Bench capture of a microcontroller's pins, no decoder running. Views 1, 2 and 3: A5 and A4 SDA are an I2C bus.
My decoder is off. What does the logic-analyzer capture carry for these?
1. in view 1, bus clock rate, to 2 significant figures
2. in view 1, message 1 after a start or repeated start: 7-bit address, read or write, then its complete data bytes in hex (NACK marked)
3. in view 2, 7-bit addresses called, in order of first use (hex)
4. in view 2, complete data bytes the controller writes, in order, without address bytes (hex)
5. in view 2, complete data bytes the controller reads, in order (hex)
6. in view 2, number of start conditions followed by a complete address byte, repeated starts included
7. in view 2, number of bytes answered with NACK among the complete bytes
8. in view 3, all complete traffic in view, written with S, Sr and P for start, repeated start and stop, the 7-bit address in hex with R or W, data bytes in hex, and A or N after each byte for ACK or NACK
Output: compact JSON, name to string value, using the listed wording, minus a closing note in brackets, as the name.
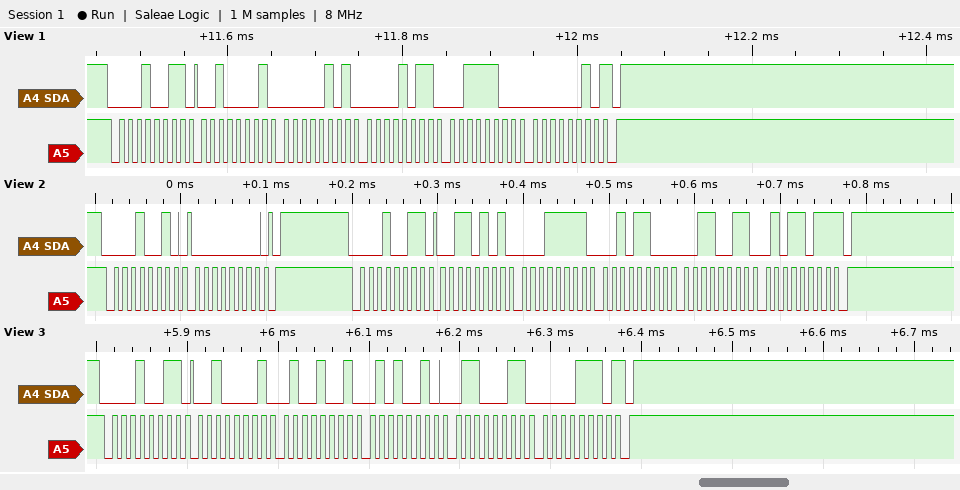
{"in view 1, bus clock rate, to 2 significant figures": "100 kHz", "in view 1, message 1 after a start or repeated start: 7-bit address, read or write, then its complete data bytes in hex": "0x09 read: 21 05 0B 3C 02 NACK", "in view 2, 7-bit addresses called, in order of first use": "0x09", "in view 2, complete data bytes the controller writes, in order, without address bytes": "00", "in view 2, complete data bytes the controller reads, in order": "35 1F 2C 33 5B", "in view 2, number of start conditions followed by a complete address byte, repeated starts included": "2", "in view 2, number of bytes answered with NACK among the complete bytes": "1", "in view 3, all complete traffic in view, written with S, Sr and P for start, repeated start and stop, the 7-bit address in hex with R or W, data bytes in hex, and A or N after each byte for ACK or NACK": "S 09R A 21 A 49 A 52 A 63 A 0E N P"}
